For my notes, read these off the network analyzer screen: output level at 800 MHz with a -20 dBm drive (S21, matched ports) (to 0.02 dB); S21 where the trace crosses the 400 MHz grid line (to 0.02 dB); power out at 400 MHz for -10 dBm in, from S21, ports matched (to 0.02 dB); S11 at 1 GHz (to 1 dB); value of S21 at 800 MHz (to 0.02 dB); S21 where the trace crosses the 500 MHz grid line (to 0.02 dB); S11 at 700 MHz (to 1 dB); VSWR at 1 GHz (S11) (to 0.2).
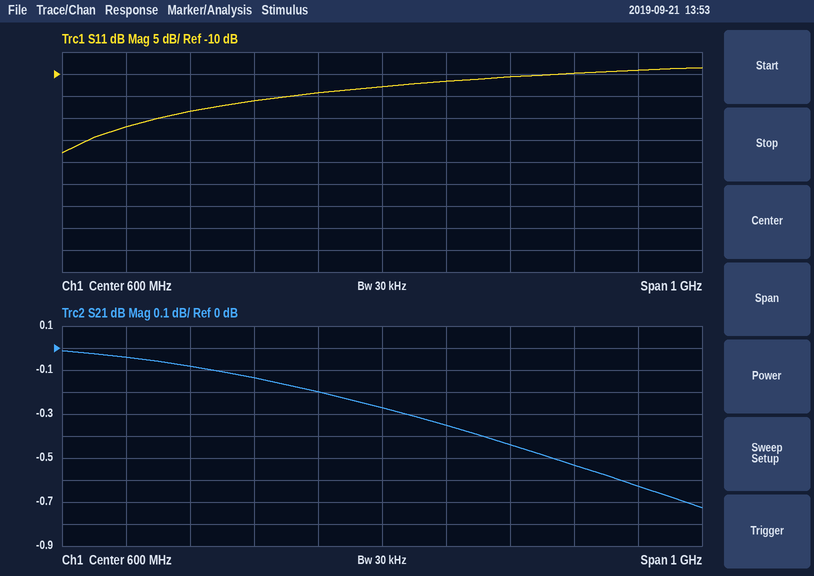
-20.44 dBm
-0.14 dB
-10.14 dBm
-9 dB
-0.44 dB
-0.20 dB
-12 dB
2.0
